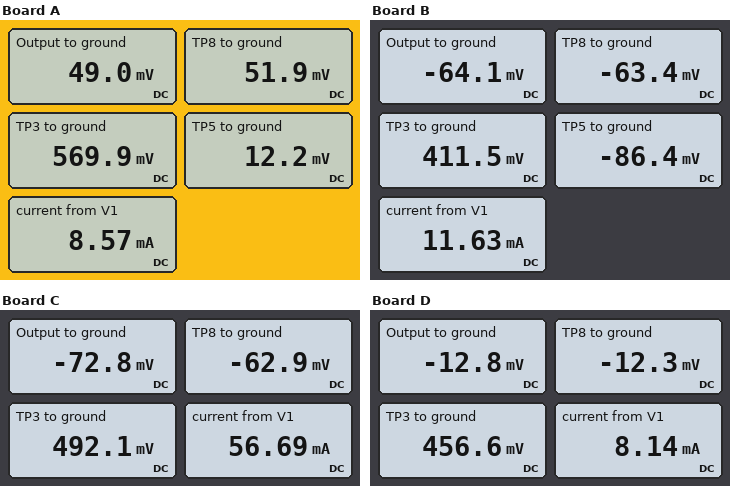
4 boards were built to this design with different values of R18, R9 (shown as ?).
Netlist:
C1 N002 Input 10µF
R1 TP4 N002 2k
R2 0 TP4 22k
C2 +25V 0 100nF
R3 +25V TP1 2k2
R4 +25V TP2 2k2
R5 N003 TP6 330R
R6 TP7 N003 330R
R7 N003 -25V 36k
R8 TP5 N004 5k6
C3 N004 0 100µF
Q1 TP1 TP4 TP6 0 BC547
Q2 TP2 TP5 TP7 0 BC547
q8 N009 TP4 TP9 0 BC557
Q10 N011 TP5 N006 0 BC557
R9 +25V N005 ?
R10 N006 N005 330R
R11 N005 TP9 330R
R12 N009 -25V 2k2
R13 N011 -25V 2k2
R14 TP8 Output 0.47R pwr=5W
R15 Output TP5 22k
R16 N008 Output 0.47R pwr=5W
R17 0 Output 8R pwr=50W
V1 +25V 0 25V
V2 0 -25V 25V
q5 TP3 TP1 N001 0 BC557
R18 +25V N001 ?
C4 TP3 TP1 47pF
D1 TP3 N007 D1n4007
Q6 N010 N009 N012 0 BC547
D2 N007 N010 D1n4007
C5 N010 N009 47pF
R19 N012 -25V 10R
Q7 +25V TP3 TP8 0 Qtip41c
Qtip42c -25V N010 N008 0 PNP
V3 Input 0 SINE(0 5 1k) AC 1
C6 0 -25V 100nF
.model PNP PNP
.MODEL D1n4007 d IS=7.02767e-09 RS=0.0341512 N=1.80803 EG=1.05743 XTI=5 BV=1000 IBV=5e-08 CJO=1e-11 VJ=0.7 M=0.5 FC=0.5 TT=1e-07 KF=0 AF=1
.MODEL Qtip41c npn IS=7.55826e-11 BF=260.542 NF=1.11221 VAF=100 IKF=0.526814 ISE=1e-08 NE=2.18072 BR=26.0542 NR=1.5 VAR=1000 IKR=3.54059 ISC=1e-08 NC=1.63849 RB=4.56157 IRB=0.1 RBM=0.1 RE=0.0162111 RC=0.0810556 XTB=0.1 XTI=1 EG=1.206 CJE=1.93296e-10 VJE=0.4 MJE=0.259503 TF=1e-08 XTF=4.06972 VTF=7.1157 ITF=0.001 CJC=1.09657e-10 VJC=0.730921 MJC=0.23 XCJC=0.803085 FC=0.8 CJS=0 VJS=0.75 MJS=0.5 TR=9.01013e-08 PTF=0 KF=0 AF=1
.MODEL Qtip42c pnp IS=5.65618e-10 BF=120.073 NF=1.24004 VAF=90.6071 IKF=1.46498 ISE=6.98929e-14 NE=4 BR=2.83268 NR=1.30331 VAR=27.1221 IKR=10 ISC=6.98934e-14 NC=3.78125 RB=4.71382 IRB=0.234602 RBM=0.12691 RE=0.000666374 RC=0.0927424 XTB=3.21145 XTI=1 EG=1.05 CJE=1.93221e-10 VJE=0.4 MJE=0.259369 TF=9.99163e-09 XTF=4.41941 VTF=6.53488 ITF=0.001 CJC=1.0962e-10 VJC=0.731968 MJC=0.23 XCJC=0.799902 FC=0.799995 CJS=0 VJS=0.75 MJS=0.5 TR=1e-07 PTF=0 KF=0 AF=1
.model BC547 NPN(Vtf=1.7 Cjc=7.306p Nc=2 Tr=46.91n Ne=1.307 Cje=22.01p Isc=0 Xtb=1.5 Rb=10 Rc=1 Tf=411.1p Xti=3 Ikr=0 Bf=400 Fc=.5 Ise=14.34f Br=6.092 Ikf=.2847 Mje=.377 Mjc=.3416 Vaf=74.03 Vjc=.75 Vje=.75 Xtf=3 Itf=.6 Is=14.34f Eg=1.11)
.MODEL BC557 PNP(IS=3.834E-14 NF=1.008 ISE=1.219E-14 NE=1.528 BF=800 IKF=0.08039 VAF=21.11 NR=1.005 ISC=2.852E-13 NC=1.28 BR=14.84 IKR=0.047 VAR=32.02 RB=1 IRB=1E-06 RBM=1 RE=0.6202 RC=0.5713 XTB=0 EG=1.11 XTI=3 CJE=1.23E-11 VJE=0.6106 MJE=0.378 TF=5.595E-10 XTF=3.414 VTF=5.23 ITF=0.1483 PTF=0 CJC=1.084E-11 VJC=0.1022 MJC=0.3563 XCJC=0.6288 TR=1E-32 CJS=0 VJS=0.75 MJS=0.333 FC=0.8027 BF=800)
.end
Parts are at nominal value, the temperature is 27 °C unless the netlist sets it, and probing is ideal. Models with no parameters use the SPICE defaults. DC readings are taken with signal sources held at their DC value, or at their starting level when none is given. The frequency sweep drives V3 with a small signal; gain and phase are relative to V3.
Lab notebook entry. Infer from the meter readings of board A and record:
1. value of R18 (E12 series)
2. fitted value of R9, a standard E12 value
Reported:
12 Ω
47 kΩ
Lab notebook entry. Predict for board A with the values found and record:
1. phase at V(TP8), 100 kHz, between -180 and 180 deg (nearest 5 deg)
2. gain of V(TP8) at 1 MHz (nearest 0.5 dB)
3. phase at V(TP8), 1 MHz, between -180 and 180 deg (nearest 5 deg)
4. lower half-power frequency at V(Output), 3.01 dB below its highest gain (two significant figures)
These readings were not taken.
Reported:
-15 deg
4.5 dB
-120 deg
760 mHz
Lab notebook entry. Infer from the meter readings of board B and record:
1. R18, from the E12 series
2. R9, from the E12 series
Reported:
22 Ω
27 kΩ
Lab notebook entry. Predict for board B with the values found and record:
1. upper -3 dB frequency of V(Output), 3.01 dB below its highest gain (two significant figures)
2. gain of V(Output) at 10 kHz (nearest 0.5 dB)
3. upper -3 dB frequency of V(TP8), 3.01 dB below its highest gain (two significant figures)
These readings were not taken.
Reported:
800 kHz
13.0 dB
800 kHz
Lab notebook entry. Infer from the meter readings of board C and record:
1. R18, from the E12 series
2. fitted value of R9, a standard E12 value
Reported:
3.3 Ω
18 kΩ
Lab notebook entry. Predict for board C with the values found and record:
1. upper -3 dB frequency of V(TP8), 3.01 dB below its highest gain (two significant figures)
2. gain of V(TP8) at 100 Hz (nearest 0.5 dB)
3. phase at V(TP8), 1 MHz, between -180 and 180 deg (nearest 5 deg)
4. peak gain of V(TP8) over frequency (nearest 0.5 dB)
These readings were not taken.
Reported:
1.0 MHz
13.5 dB
-85 deg
13.5 dB
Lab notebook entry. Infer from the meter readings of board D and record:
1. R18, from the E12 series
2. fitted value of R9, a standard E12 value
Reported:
18 Ω
33 kΩ
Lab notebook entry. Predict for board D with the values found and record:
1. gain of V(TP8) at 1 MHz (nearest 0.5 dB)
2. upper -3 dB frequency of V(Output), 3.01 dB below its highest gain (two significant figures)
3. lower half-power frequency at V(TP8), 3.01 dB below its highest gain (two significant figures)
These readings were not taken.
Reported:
5.0 dB
520 kHz
760 mHz
